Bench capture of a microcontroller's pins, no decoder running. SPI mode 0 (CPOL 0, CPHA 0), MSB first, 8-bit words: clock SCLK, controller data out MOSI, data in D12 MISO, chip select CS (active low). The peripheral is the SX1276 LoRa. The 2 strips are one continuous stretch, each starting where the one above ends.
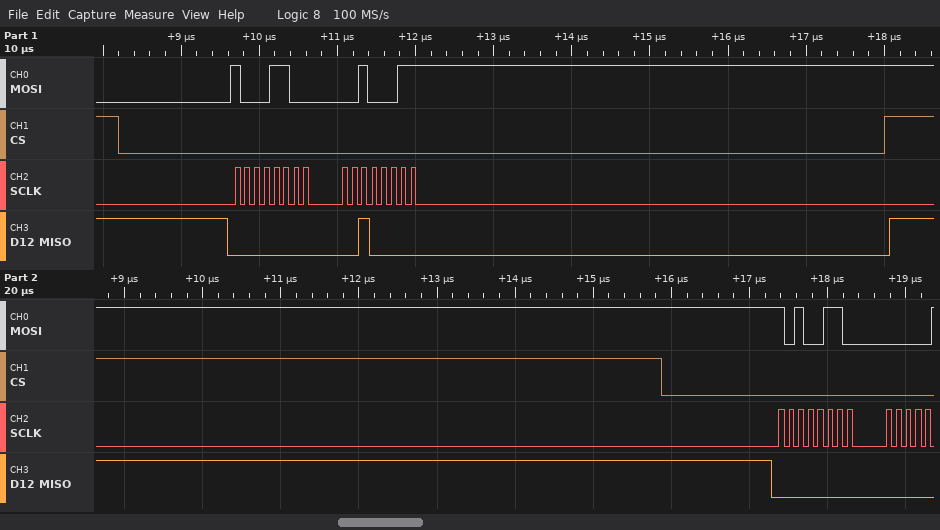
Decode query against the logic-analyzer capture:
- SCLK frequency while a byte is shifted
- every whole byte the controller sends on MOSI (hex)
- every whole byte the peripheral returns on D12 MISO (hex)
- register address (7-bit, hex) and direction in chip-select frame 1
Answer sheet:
8 MHz
0x8C 0x23 0xA6
0x00 0x20 0x00
0x0C write
